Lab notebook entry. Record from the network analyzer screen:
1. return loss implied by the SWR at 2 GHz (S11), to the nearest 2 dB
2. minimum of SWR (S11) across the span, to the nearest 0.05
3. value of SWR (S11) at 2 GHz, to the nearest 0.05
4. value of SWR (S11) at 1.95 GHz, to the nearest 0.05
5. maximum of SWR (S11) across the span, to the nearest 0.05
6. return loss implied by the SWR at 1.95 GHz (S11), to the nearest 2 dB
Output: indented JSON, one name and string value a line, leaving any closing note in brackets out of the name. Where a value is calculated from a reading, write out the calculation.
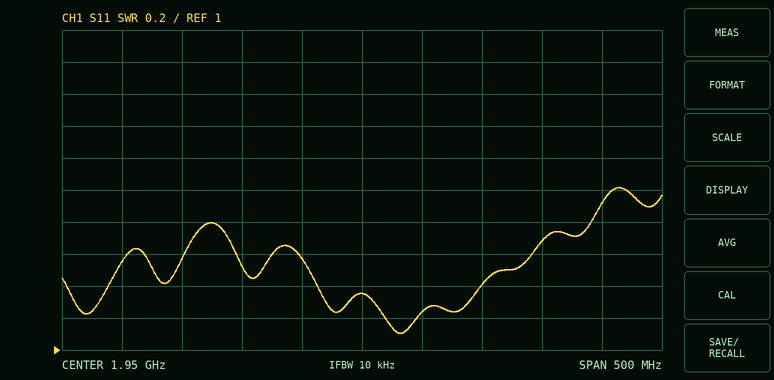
{
  "return loss implied by the SWR at 2 GHz (S11), to the nearest 2 dB": "−20 log10((1.25 − 1)/(1.25 + 1)) ≈ 19.1 dB, so 20 dB to the nearest 2 dB",
  "minimum of SWR (S11) across the span, to the nearest 0.05": "1.10",
  "value of SWR (S11) at 2 GHz, to the nearest 0.05": "1.25",
  "value of SWR (S11) at 1.95 GHz, to the nearest 0.05": "1.35",
  "maximum of SWR (S11) across the span, to the nearest 0.05": "2.00",
  "return loss implied by the SWR at 1.95 GHz (S11), to the nearest 2 dB": "−20 log10((1.35 − 1)/(1.35 + 1)) ≈ 16 dB"
}
